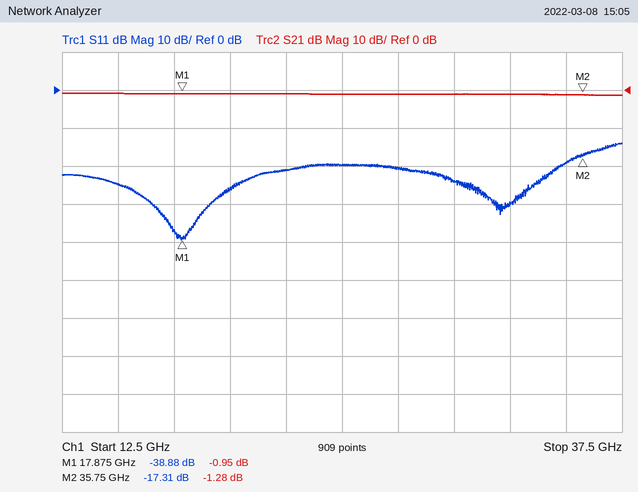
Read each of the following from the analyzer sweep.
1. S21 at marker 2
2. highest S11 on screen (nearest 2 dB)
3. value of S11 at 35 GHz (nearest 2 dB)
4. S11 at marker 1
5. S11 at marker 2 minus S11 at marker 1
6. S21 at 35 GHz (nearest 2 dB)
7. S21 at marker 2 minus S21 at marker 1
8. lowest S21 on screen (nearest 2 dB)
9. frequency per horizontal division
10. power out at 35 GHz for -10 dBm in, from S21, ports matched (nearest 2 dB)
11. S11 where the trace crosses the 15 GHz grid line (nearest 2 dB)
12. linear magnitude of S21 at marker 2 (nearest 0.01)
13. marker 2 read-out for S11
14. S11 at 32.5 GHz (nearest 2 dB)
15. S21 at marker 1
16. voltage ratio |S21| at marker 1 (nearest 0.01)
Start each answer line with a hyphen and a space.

- -1.28 dB
- -14 dB
- -20 dB
- -38.88 dB
- 21.57 dB
- -2 dB
- -0.33 dB
- -2 dB
- 2.5 GHz
- -12 dBm
- -24 dB
- 0.86
- -17.31 dB
- -30 dB
- -0.95 dB
- 0.90
